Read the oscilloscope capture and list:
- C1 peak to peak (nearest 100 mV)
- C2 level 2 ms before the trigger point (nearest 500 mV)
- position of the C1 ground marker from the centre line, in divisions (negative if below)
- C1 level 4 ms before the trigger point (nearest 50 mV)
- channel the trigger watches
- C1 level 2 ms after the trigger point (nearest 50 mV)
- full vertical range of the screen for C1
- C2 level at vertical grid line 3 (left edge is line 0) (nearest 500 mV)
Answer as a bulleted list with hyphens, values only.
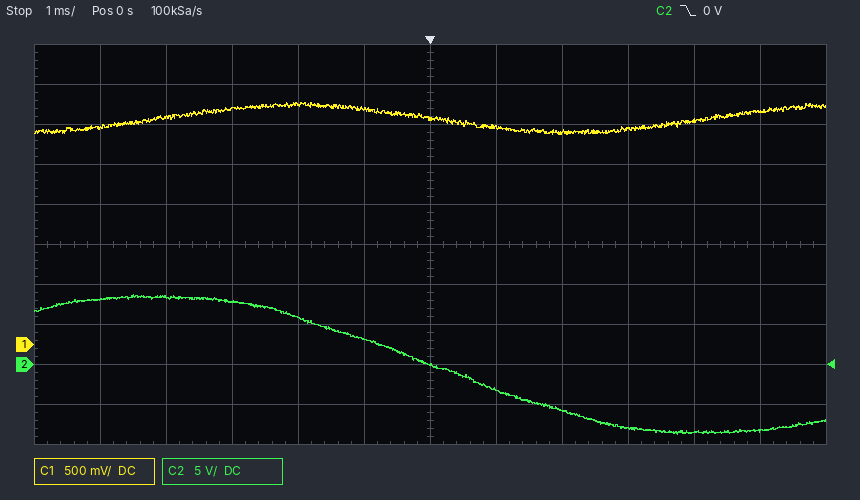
- 400 mV
- 6.0 V
- -2.5 div
- 2.85 V
- C2
- 2.65 V
- 5 V
- 8.0 V
